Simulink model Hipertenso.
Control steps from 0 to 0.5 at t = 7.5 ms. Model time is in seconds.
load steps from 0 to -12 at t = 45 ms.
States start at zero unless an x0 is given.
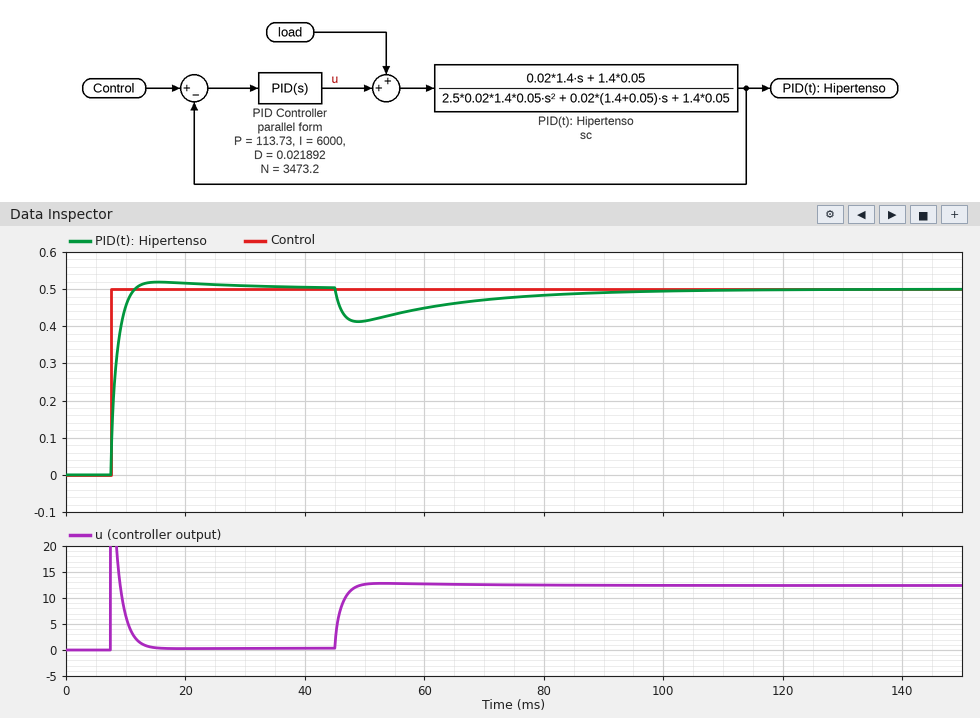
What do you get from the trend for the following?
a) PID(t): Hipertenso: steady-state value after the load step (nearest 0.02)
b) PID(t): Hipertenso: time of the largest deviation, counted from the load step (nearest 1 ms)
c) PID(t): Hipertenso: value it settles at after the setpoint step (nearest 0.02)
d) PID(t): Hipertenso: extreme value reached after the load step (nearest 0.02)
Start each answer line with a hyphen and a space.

- 0.50
- 4 ms
- 0.50
- 0.42
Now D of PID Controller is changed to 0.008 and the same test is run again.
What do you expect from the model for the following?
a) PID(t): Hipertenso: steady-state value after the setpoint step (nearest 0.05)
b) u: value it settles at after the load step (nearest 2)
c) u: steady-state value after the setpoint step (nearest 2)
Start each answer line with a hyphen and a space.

- 0.50
- 12
- 0
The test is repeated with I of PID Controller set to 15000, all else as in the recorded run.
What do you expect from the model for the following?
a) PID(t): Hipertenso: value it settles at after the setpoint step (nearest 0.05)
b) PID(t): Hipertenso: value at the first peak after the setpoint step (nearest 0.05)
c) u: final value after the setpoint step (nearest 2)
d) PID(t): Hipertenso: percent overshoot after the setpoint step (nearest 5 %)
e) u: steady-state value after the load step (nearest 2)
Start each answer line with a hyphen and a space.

- 0.50
- 0.55
- 0
- 10 %
- 12
